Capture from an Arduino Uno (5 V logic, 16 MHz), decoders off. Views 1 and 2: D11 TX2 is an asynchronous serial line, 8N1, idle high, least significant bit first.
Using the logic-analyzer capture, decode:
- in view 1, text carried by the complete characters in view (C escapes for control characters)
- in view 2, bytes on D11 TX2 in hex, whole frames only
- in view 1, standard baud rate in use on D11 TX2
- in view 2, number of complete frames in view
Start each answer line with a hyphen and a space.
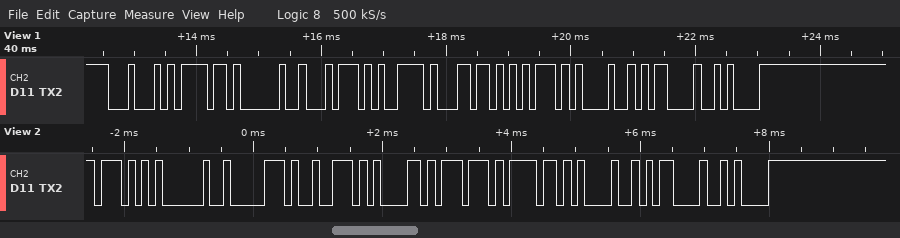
- "Do tylu!\r\n"
- 57 20 70 72 61 77 6F 21 0D 0A
- 9600 baud
- 10
